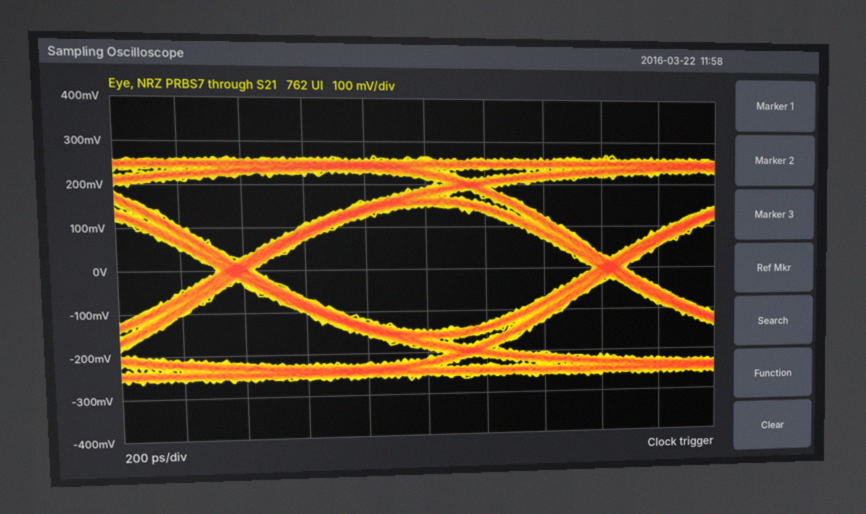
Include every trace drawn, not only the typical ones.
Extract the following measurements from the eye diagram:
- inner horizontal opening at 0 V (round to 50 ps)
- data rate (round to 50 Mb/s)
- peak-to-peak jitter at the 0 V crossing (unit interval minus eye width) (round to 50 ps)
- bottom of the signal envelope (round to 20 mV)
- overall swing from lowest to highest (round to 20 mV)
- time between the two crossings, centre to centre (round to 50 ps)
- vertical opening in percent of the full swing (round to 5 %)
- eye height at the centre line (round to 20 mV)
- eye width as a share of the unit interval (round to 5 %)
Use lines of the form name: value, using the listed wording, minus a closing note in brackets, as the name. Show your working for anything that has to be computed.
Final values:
inner horizontal opening at 0 V: 1.15 ns
data rate: 800 Mb/s
peak-to-peak jitter at the 0 V crossing (unit interval minus eye width): 100 ps
bottom of the signal envelope: -260 mV
overall swing from lowest to highest: 540 mV
time between the two crossings, centre to centre: 1.25 ns
vertical opening in percent of the full swing: 300 mV / 540 mV ≈ 55.6 %, so 55 % to the nearest 5 %
eye height at the centre line: 300 mV
eye width as a share of the unit interval: 1.15 ns / 1.25 ns ≈ 92.0 %, so 90 % to the nearest 5 %
